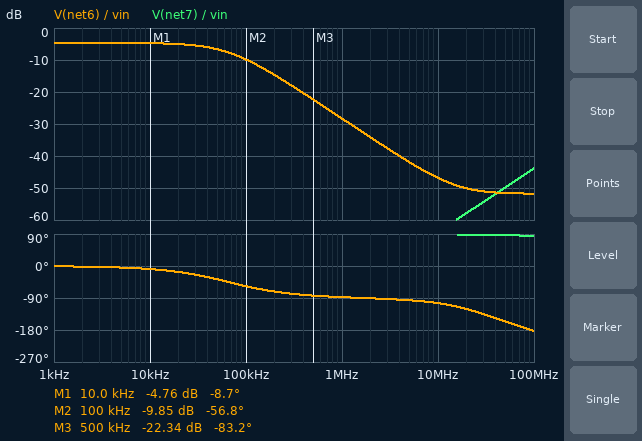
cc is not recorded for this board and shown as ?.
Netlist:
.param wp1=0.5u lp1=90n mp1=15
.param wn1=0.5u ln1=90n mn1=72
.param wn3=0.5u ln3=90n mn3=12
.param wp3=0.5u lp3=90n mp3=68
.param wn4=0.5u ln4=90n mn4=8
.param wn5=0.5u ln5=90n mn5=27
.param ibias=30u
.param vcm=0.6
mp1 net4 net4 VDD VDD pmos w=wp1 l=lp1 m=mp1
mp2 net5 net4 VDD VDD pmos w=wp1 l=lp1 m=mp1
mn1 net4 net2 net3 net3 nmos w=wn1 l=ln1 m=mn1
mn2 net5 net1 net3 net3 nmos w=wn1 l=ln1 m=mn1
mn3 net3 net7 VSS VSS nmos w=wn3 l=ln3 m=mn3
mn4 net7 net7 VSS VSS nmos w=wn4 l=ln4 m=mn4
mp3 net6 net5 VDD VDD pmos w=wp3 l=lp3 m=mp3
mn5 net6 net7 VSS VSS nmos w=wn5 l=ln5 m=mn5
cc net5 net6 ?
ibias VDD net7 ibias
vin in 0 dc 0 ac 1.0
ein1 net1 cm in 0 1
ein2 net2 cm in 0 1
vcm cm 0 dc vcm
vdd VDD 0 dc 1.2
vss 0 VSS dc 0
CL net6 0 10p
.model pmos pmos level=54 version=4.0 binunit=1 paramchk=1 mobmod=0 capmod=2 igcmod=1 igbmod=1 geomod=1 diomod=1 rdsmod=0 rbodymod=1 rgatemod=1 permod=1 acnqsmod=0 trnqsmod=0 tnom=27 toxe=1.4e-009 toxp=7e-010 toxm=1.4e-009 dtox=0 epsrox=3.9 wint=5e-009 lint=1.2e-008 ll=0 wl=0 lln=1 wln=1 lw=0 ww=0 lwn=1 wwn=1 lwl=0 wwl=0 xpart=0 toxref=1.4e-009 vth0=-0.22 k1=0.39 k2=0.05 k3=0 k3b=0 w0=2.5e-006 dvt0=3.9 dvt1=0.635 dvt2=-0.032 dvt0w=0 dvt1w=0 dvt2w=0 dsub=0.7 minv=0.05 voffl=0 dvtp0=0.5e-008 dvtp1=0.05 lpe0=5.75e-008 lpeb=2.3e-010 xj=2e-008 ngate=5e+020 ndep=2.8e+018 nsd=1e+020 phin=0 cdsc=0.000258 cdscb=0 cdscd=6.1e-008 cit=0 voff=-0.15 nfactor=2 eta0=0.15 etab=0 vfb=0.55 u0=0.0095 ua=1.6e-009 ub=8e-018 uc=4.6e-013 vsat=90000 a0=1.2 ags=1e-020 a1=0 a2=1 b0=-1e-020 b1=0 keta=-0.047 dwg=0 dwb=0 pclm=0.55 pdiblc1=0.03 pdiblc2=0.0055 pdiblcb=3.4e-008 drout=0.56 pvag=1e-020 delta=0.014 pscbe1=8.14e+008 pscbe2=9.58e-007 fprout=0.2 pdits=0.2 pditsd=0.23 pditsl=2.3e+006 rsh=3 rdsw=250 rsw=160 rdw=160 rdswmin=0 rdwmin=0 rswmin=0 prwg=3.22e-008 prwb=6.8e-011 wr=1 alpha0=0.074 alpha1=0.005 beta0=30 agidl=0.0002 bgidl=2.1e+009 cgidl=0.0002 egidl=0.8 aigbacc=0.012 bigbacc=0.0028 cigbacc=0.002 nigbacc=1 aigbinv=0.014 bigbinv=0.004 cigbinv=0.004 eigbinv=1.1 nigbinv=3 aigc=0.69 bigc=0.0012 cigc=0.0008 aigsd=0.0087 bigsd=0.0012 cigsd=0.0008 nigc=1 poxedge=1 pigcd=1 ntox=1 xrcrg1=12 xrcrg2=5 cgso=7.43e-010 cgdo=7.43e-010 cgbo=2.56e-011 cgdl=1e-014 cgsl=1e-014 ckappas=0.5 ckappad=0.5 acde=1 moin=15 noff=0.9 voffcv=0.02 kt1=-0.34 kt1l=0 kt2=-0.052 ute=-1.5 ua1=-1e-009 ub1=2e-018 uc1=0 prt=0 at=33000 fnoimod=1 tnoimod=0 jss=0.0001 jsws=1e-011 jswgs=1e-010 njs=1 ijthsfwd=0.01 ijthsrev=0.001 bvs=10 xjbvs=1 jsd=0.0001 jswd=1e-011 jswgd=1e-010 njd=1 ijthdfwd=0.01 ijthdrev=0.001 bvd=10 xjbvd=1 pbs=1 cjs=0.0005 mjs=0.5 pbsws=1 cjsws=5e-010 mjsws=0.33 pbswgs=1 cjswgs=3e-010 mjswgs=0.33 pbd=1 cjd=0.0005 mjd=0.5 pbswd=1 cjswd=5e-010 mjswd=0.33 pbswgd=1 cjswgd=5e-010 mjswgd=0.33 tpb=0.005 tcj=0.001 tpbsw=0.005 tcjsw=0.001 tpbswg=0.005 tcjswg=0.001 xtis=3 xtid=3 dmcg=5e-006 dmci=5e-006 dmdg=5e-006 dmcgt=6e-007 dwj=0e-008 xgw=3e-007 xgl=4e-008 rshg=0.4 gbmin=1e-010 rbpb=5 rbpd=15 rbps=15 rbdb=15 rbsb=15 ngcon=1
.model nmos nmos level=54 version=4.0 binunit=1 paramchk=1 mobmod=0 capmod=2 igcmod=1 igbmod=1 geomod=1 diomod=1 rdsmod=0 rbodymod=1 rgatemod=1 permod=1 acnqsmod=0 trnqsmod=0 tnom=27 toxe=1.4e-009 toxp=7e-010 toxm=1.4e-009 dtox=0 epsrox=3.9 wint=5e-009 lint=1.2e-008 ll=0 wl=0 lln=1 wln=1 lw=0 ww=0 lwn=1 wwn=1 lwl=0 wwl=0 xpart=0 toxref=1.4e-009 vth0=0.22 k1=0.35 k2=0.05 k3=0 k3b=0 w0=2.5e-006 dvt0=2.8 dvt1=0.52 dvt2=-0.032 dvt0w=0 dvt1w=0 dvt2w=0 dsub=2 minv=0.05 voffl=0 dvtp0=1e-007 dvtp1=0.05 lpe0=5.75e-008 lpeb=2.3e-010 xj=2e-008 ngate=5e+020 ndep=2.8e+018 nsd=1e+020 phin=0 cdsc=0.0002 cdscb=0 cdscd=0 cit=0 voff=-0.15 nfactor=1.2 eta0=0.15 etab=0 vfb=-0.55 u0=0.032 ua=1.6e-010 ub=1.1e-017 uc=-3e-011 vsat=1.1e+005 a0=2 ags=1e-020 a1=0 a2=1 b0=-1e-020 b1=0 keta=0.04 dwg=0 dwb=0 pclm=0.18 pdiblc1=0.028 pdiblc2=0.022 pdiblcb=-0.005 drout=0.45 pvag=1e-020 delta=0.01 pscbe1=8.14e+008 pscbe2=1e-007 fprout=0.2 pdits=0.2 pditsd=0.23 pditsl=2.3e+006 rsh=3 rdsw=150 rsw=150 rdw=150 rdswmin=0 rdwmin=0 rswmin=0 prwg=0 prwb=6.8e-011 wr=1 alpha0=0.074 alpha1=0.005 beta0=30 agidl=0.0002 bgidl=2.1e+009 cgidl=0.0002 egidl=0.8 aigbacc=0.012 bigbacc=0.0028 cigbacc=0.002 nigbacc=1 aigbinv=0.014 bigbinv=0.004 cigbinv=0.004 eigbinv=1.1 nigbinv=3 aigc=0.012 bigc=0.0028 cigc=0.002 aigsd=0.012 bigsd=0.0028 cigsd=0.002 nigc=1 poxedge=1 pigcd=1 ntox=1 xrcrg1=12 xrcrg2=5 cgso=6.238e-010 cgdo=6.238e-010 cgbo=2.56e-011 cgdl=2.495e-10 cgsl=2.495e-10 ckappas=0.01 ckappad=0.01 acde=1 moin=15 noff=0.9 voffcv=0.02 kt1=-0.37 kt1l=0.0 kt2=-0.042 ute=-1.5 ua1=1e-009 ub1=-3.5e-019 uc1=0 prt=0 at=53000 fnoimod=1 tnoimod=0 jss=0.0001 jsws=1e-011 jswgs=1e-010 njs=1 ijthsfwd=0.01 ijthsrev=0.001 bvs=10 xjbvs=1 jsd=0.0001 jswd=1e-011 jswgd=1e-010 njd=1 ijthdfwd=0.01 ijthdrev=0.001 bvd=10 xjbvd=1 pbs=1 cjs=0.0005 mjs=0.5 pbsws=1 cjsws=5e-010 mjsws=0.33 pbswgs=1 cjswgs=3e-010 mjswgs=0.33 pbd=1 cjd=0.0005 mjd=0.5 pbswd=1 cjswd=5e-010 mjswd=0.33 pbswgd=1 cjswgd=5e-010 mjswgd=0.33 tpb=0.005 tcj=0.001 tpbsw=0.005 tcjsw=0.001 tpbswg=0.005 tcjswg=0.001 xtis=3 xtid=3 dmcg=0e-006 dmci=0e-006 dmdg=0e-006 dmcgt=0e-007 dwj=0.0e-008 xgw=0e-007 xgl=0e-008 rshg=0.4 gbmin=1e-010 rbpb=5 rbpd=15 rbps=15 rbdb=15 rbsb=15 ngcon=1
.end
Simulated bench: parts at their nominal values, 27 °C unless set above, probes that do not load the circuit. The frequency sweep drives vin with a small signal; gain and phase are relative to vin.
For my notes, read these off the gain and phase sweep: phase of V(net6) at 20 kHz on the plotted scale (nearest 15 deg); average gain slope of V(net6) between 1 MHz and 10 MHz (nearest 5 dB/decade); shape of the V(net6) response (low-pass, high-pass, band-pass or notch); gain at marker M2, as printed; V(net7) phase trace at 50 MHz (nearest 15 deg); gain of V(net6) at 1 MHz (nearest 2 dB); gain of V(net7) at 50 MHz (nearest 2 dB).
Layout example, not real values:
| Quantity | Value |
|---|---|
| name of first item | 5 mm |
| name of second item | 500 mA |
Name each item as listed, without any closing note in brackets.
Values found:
| Quantity | Value |
|---|---|
| phase of V(net6) at 20 kHz on the plotted scale | -15 deg |
| average gain slope of V(net6) between 1 MHz and 10 MHz | -20 dB/decade |
| shape of the V(net6) response | low-pass |
| gain at marker M2, as printed | -9.85 dB |
| V(net7) phase trace at 50 MHz | 90 deg |
| gain of V(net6) at 1 MHz | -28 dB |
| gain of V(net7) at 50 MHz | -50 dB |
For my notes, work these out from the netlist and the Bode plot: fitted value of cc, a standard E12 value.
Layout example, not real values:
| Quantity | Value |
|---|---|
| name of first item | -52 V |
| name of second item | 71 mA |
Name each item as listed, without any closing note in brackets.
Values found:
| Quantity | Value |
|---|---|
| fitted value of cc, a standard E12 value | 2.7 pF |
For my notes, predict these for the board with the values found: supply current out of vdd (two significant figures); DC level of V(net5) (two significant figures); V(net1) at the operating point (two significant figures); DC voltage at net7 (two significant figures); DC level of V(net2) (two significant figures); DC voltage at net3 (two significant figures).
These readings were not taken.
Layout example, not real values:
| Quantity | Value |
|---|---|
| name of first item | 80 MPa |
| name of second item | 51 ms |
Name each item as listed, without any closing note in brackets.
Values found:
| Quantity | Value |
|---|---|
| supply current out of vdd | 180 µA |
| DC level of V(net5) | 820 mV |
| V(net1) at the operating point | 600 mV |
| DC voltage at net7 | 390 mV |
| DC level of V(net2) | 600 mV |
| DC voltage at net3 | 340 mV |
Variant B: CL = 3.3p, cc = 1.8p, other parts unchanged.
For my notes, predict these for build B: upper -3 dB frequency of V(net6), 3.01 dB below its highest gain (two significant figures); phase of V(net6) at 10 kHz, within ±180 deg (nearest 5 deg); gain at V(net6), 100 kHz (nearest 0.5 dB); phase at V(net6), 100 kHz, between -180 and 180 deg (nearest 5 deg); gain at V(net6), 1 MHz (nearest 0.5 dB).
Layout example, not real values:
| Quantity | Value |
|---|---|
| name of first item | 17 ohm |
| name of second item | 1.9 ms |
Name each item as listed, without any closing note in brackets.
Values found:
| Quantity | Value |
|---|---|
| upper -3 dB frequency of V(net6), 3.01 dB below its highest gain | 100 kHz |
| phase of V(net6) at 10 kHz, within ±180 deg | -5 deg |
| gain at V(net6), 100 kHz | -7.5 dB |
| phase at V(net6), 100 kHz, between -180 and 180 deg | -45 deg |
| gain at V(net6), 1 MHz | -24.5 dB |
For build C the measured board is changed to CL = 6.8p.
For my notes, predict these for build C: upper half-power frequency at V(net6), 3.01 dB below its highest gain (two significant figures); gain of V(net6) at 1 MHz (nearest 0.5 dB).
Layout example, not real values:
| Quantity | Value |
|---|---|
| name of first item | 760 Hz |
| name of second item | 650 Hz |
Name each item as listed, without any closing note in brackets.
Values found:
| Quantity | Value |
|---|---|
| upper half-power frequency at V(net6), 3.01 dB below its highest gain | 67 kHz |
| gain of V(net6) at 1 MHz | -28.0 dB |
